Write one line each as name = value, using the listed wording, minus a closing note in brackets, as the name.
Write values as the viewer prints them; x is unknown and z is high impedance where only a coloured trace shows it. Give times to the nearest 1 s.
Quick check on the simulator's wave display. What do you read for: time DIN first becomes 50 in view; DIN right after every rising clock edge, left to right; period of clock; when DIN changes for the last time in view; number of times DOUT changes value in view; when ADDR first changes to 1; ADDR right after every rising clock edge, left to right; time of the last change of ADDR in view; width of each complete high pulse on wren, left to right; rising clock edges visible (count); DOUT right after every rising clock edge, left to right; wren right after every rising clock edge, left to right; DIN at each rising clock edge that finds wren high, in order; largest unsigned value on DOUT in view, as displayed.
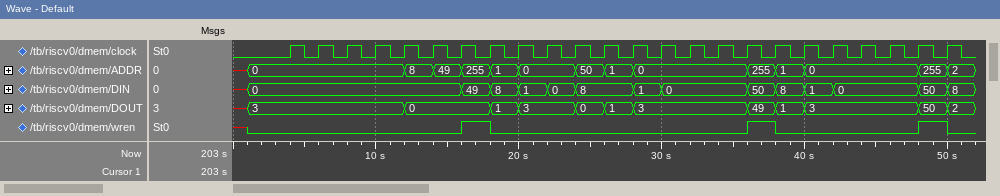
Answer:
time DIN first becomes 50 in view = 36 s
DIN right after every rising clock edge, left to right = 0, 0, 0, 0, 0, 0, 49, 8, 1, 0, 8, 8, 1, 0, 0, 0, 50, 8, 1, 0, 0, 0, 50, 8
period of clock = 2 s
when DIN changes for the last time in view = 50 s
number of times DOUT changes value in view = 12
when ADDR first changes to 1 = 18 s
ADDR right after every rising clock edge, left to right = 0, 0, 0, 0, 8, 49, 255, 1, 0, 0, 50, 1, 0, 0, 0, 0, 255, 1, 0, 0, 0, 0, 255, 2
time of the last change of ADDR in view = 50 s
width of each complete high pulse on wren, left to right = 2 s, 2 s, 2 s
rising clock edges visible = 24
DOUT right after every rising clock edge, left to right = 3, 3, 3, 3, 0, 0, 0, 1, 3, 3, 0, 1, 3, 3, 3, 3, 49, 1, 3, 3, 3, 3, 50, 2
wren right after every rising clock edge, left to right = 0 0 0 0 0 0 1 0 0 0 0 0 0 0 0 0 1 0 0 0 0 0 1 0
DIN at each rising clock edge that finds wren high, in order = 49, 50, 50
largest unsigned value on DOUT in view, as displayed = 50
